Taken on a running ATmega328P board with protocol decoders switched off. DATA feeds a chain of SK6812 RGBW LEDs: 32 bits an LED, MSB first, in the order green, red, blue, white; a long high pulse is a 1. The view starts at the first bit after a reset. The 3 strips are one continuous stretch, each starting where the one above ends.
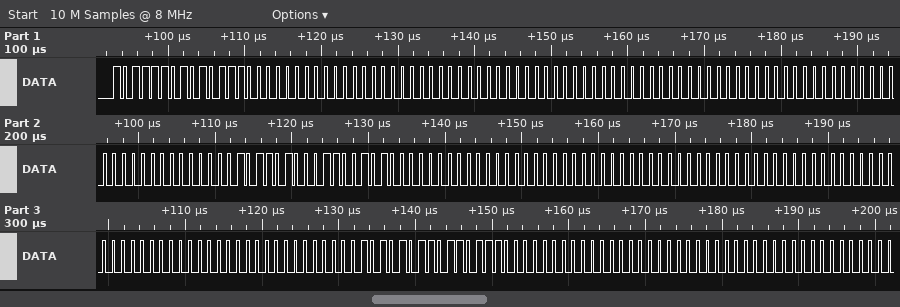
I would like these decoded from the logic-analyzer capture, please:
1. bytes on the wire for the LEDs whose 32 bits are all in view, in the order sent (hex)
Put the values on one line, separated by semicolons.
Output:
BD 5C 00 00 00 00 00 00 00 00 00 00 B4 65 00 00 00 00 00 00 00 00 00 00 AB 6E 00 00
